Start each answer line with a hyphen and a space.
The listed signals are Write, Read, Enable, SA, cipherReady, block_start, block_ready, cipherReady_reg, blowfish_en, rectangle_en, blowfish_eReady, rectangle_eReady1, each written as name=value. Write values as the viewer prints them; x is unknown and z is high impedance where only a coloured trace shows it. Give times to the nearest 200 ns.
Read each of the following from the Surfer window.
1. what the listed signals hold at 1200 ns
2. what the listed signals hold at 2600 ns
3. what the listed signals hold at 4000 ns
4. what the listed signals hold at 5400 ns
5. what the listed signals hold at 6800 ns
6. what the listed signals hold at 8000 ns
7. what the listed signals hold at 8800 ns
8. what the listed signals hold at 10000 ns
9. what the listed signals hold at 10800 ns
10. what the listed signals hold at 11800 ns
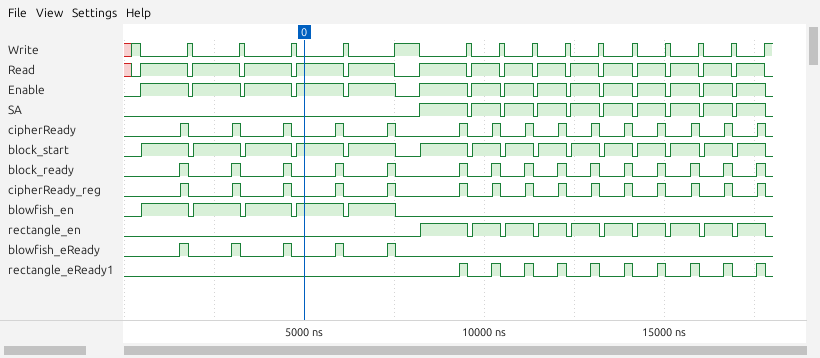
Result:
- Write=0, Read=1, Enable=1, SA=0, cipherReady=0, block_start=1, block_ready=0, cipherReady_reg=0, blowfish_en=1, rectangle_en=0, blowfish_eReady=0, rectangle_eReady1=0
- Write=0, Read=1, Enable=1, SA=0, cipherReady=0, block_start=1, block_ready=0, cipherReady_reg=0, blowfish_en=1, rectangle_en=0, blowfish_eReady=0, rectangle_eReady1=0
- Write=0, Read=1, Enable=1, SA=0, cipherReady=0, block_start=1, block_ready=0, cipherReady_reg=0, blowfish_en=1, rectangle_en=0, blowfish_eReady=0, rectangle_eReady1=0
- Write=0, Read=1, Enable=1, SA=0, cipherReady=0, block_start=1, block_ready=0, cipherReady_reg=0, blowfish_en=1, rectangle_en=0, blowfish_eReady=0, rectangle_eReady1=0
- Write=0, Read=1, Enable=1, SA=0, cipherReady=0, block_start=1, block_ready=0, cipherReady_reg=0, blowfish_en=1, rectangle_en=0, blowfish_eReady=0, rectangle_eReady1=0
- Write=1, Read=0, Enable=0, SA=0, cipherReady=0, block_start=0, block_ready=0, cipherReady_reg=0, blowfish_en=0, rectangle_en=0, blowfish_eReady=0, rectangle_eReady1=0
- Write=0, Read=1, Enable=1, SA=1, cipherReady=0, block_start=1, block_ready=0, cipherReady_reg=0, blowfish_en=0, rectangle_en=1, blowfish_eReady=0, rectangle_eReady1=0
- Write=0, Read=1, Enable=1, SA=1, cipherReady=0, block_start=1, block_ready=0, cipherReady_reg=0, blowfish_en=0, rectangle_en=1, blowfish_eReady=0, rectangle_eReady1=0
- Write=0, Read=1, Enable=1, SA=1, cipherReady=0, block_start=1, block_ready=0, cipherReady_reg=0, blowfish_en=0, rectangle_en=1, blowfish_eReady=0, rectangle_eReady1=0
- Write=0, Read=1, Enable=1, SA=1, cipherReady=0, block_start=1, block_ready=0, cipherReady_reg=0, blowfish_en=0, rectangle_en=1, blowfish_eReady=0, rectangle_eReady1=0
